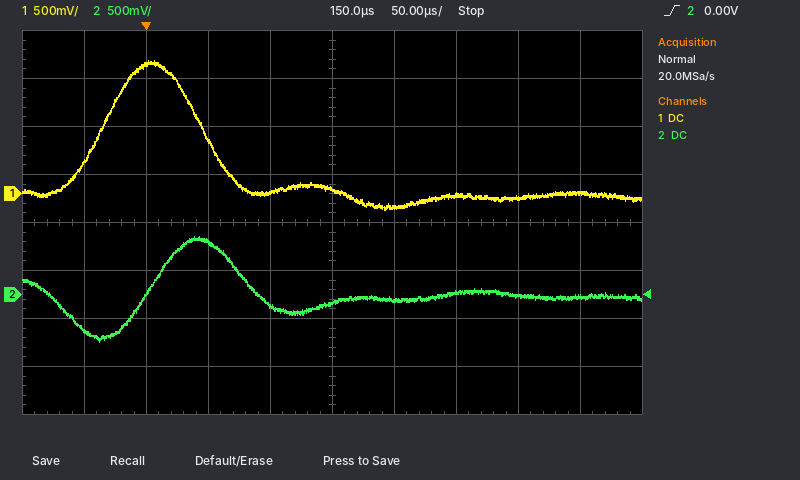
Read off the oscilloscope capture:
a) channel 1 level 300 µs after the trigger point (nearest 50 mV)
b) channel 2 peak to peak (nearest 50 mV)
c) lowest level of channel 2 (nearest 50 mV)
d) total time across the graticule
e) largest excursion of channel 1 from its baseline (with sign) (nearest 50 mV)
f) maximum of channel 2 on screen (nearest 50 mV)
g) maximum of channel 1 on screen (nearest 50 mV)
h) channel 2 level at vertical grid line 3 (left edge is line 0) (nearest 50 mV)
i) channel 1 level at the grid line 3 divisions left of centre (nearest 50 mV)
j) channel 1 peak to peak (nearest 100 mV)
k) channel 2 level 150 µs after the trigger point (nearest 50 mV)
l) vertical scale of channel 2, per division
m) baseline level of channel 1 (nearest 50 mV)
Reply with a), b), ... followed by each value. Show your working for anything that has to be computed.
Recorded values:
a) -50 mV
b) 600 mV − (-500 mV) = 1.10 V
c) -500 mV
d) 500 µs
e) 1.40 V − (0 mV) = +1.40 V
f) 600 mV
g) 1.40 V
h) 550 mV
i) 1.35 V
j) 1.60 V
k) -100 mV
l) 500 mV
m) 0 mV
